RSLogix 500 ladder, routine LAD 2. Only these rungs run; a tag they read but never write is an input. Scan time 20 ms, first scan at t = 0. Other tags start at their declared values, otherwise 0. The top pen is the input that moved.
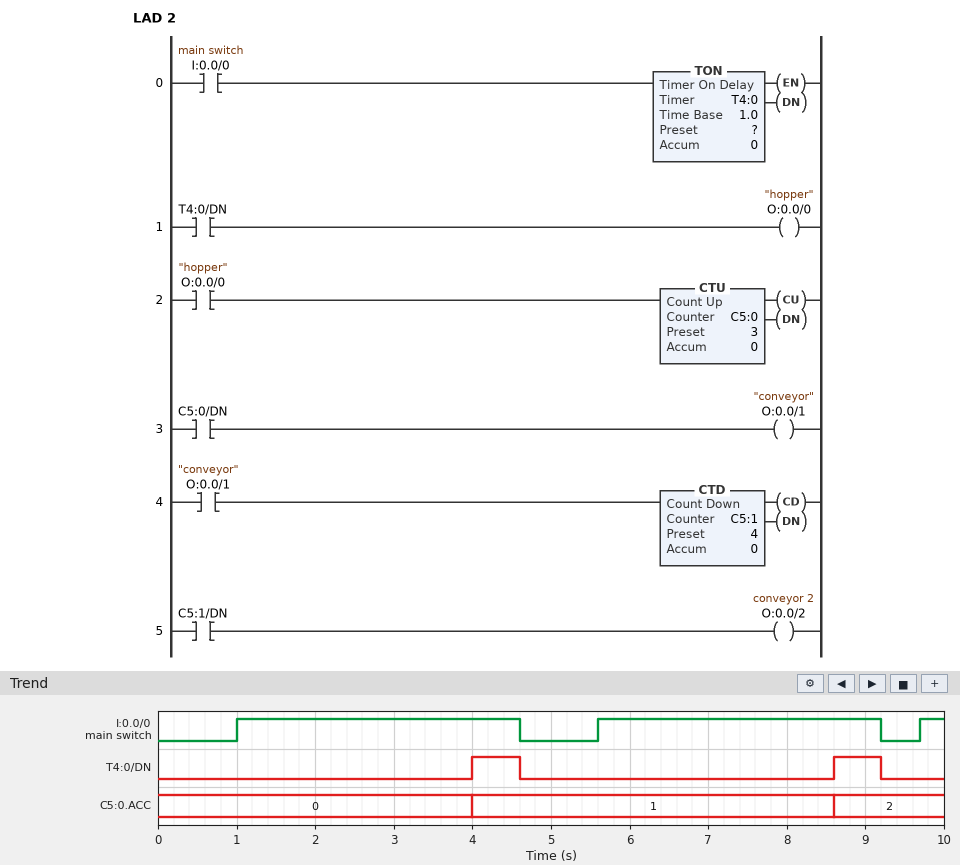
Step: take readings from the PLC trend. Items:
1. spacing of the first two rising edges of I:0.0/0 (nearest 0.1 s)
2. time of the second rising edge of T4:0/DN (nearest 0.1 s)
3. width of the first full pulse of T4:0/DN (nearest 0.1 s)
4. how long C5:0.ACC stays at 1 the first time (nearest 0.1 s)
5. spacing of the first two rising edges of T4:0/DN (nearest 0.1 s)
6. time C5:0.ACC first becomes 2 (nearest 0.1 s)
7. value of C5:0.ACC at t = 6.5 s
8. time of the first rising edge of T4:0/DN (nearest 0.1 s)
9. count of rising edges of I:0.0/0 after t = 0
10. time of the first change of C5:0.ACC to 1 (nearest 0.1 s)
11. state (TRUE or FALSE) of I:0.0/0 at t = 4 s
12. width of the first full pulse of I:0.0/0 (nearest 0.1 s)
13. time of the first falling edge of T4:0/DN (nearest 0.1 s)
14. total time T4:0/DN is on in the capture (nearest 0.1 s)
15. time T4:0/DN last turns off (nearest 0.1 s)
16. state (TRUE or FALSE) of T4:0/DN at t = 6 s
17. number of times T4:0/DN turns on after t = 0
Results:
4.6 s
8.6 s
0.6 s
4.6 s
4.6 s
8.6 s
1
4.0 s
3
4.0 s
TRUE
3.6 s
4.6 s
1.2 s
9.2 s
FALSE
2
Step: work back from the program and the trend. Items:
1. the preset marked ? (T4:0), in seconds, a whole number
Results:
3 s
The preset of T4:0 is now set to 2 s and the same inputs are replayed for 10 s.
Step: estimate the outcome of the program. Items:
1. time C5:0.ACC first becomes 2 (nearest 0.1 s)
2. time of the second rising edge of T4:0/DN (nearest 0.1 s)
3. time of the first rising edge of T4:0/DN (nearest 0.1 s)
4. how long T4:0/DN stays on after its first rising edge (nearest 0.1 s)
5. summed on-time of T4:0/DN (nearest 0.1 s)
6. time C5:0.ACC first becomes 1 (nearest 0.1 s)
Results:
7.6 s
7.6 s
3.0 s
1.6 s
3.2 s
3.0 s
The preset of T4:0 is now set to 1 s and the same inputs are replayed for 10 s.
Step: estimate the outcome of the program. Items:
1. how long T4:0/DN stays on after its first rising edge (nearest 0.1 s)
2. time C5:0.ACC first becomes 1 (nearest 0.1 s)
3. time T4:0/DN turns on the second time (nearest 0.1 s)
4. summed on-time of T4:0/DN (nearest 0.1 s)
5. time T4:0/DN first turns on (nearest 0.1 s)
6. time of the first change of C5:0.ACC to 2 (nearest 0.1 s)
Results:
2.6 s
2.0 s
6.6 s
5.2 s
2.0 s
6.6 s
